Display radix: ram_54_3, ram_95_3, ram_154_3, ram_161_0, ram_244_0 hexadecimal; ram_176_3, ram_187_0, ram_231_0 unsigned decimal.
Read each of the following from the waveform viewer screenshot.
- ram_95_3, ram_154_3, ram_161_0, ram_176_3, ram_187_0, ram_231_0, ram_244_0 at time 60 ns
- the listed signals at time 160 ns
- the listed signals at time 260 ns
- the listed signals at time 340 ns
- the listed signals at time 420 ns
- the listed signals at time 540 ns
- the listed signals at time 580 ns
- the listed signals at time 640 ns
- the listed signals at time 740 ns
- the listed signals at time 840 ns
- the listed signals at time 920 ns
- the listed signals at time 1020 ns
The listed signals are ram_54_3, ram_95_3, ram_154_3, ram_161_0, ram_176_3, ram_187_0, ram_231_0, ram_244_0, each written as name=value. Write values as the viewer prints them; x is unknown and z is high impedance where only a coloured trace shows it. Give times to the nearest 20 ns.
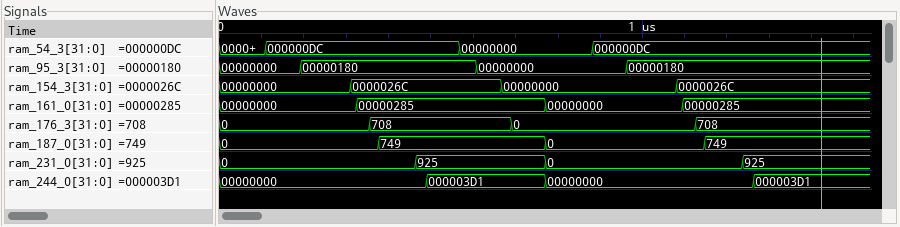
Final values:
ram_95_3=00000000, ram_154_3=00000000, ram_161_0=00000000, ram_176_3=0, ram_187_0=0, ram_231_0=0, ram_244_0=00000000
ram_54_3=000000DC, ram_95_3=00000000, ram_154_3=00000000, ram_161_0=00000000, ram_176_3=0, ram_187_0=0, ram_231_0=0, ram_244_0=00000000
ram_54_3=000000DC, ram_95_3=00000180, ram_154_3=00000000, ram_161_0=00000000, ram_176_3=0, ram_187_0=0, ram_231_0=0, ram_244_0=00000000
ram_54_3=000000DC, ram_95_3=00000180, ram_154_3=0000026C, ram_161_0=00000285, ram_176_3=0, ram_187_0=0, ram_231_0=0, ram_244_0=00000000
ram_54_3=000000DC, ram_95_3=00000180, ram_154_3=0000026C, ram_161_0=00000285, ram_176_3=708, ram_187_0=749, ram_231_0=0, ram_244_0=00000000
ram_54_3=000000DC, ram_95_3=00000180, ram_154_3=0000026C, ram_161_0=00000285, ram_176_3=708, ram_187_0=749, ram_231_0=925, ram_244_0=000003D1
ram_54_3=00000000, ram_95_3=00000180, ram_154_3=0000026C, ram_161_0=00000285, ram_176_3=708, ram_187_0=749, ram_231_0=925, ram_244_0=000003D1
ram_54_3=00000000, ram_95_3=00000000, ram_154_3=0000026C, ram_161_0=00000285, ram_176_3=708, ram_187_0=749, ram_231_0=925, ram_244_0=000003D1
ram_54_3=00000000, ram_95_3=00000000, ram_154_3=00000000, ram_161_0=00000285, ram_176_3=0, ram_187_0=749, ram_231_0=925, ram_244_0=000003D1
ram_54_3=00000000, ram_95_3=00000000, ram_154_3=00000000, ram_161_0=00000000, ram_176_3=0, ram_187_0=0, ram_231_0=0, ram_244_0=00000000
ram_54_3=000000DC, ram_95_3=00000000, ram_154_3=00000000, ram_161_0=00000000, ram_176_3=0, ram_187_0=0, ram_231_0=0, ram_244_0=00000000
ram_54_3=000000DC, ram_95_3=00000180, ram_154_3=00000000, ram_161_0=00000000, ram_176_3=0, ram_187_0=0, ram_231_0=0, ram_244_0=00000000
